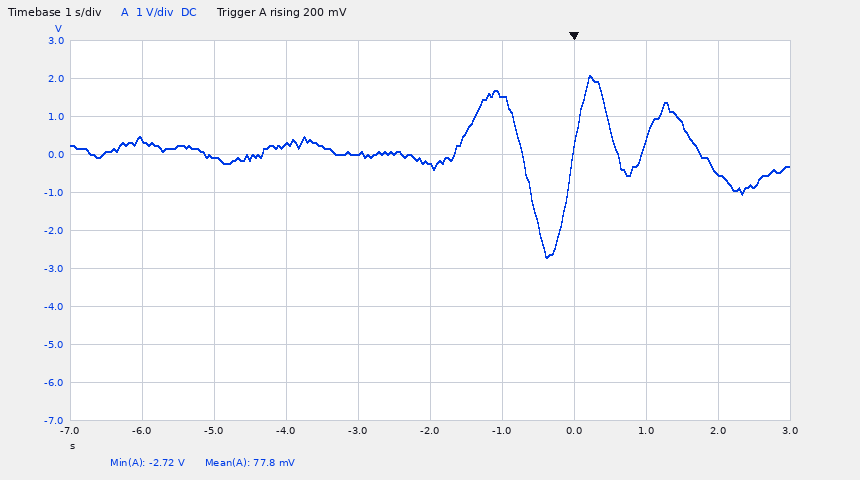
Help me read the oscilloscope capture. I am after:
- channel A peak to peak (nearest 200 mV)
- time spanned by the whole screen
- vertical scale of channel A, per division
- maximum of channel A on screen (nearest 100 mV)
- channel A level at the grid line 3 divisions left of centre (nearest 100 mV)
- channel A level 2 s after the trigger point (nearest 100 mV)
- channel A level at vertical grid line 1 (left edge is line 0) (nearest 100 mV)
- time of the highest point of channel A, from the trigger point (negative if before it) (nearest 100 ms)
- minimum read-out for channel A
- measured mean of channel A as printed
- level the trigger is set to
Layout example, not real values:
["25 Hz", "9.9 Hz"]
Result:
["4.8 V", "10 s", "1 V", "2.1 V", "-100 mV", "-500 mV", "400 mV", "+200 ms", "-2.72 V", "77.8 mV", "200 mV"]
